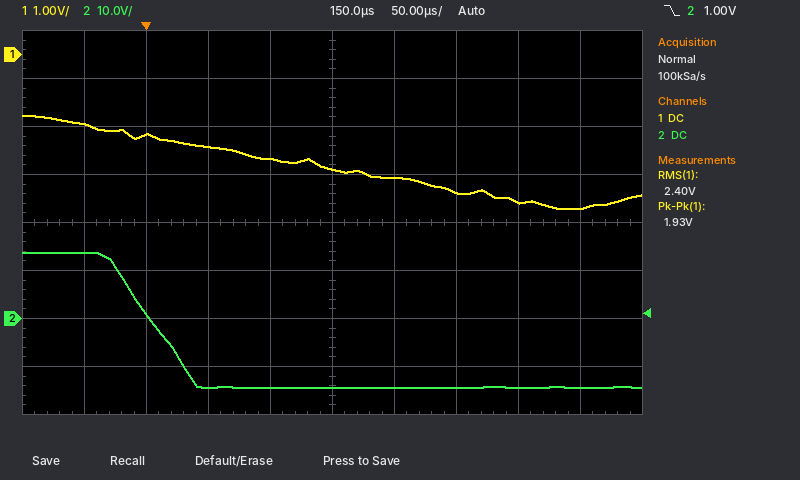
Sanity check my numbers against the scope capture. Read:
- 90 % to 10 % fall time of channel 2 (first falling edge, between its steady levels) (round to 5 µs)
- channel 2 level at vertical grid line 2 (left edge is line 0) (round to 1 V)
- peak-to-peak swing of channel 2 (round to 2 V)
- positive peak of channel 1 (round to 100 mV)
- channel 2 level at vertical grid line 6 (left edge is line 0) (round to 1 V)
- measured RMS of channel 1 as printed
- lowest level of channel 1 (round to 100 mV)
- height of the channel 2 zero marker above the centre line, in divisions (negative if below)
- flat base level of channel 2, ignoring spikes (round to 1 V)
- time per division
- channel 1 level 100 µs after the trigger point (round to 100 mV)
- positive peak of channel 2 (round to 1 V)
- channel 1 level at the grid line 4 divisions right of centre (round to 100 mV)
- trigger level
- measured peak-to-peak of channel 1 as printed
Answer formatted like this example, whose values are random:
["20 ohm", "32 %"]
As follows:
["60 µs", "1 V", "28 V", "-1.3 V", "-14 V", "2.40 V", "-3.2 V", "-2.0 div", "-14 V", "50 µs", "-2.2 V", "14 V", "-3.2 V", "1.00 V", "1.93 V"]
